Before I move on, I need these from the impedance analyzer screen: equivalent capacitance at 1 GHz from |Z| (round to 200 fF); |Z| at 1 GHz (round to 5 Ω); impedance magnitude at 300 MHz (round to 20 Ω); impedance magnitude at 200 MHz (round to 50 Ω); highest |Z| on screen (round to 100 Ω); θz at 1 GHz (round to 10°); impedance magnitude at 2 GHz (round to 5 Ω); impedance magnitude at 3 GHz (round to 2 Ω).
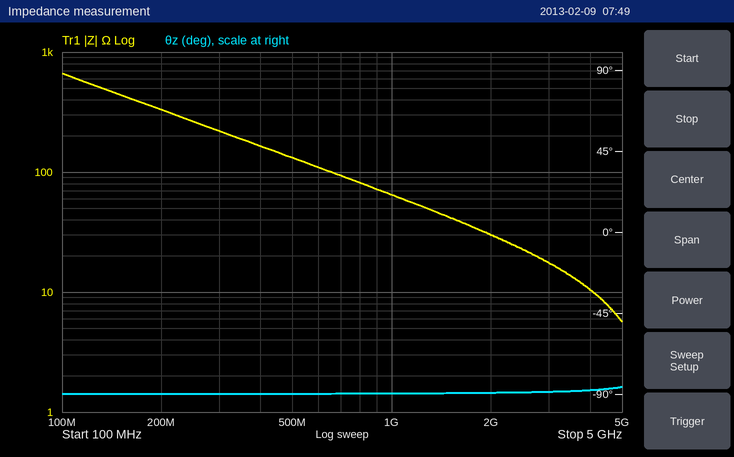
2.4 pF
65 Ω
220 Ω
350 Ω
700 Ω
-90°
30 Ω
18 Ω
